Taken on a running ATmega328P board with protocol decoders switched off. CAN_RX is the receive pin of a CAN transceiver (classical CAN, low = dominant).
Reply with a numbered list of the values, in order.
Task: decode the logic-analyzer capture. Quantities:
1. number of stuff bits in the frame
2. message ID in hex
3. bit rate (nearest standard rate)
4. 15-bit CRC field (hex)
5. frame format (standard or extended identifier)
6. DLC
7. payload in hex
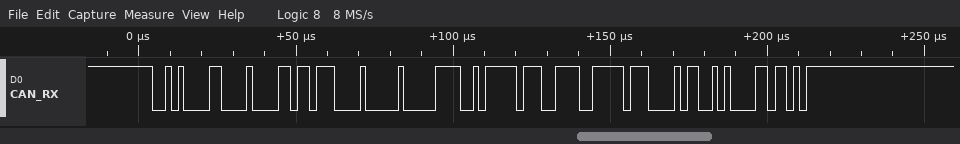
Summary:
1. 4
2. 0x286
3. 500 kbit/s
4. 0x1436
5. standard
6. 8
7. 6D C2 00 72 FF 3C FF 0B
